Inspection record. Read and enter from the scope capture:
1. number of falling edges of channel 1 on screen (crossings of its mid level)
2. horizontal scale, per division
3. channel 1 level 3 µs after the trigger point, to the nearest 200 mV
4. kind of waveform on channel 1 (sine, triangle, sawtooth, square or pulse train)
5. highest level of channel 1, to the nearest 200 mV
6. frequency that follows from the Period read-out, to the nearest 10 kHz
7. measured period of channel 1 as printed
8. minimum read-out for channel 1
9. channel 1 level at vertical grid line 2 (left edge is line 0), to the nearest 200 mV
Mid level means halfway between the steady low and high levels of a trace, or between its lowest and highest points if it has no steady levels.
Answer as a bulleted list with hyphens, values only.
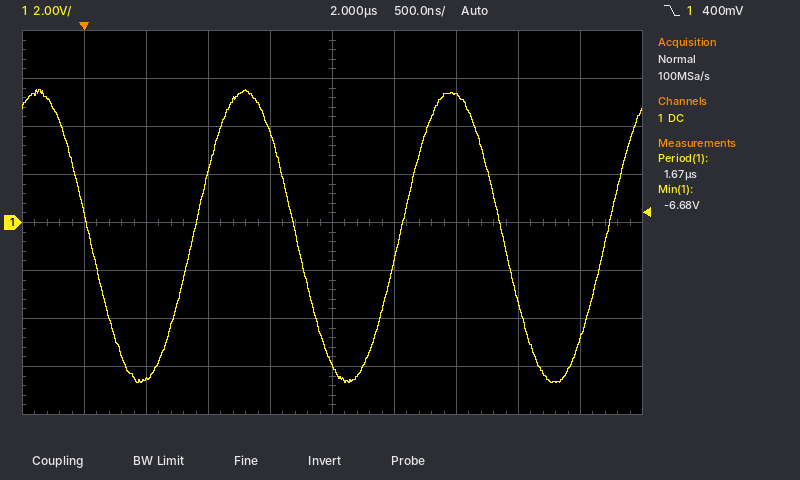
- 3
- 500 ns
- 5.4 V
- sine
- 5.6 V
- 600 kHz
- 1.67 µs
- -6.68 V
- -6.6 V
